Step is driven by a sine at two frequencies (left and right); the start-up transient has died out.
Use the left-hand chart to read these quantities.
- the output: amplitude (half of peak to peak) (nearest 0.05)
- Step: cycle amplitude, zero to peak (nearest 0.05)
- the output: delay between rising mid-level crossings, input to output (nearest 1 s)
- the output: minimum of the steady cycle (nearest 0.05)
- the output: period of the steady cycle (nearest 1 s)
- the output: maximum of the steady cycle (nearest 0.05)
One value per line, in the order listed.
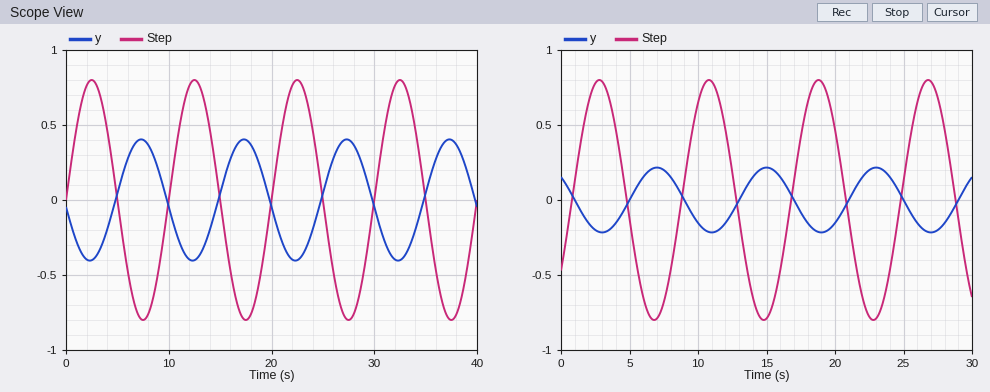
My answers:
0.40
0.80
5 s
-0.40
10 s
0.40
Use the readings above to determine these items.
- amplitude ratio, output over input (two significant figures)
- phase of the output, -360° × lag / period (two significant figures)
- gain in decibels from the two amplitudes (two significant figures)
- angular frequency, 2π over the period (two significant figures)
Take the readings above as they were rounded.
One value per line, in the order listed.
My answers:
0.50
-180°
-6.0 dB
0.63 rad/s
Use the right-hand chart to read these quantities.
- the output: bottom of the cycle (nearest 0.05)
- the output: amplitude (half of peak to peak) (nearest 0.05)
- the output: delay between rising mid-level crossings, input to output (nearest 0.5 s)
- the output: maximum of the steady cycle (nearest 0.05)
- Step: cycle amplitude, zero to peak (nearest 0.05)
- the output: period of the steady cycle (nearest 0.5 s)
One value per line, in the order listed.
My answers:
-0.20
0.20
4.0 s
0.20
0.80
8.0 s
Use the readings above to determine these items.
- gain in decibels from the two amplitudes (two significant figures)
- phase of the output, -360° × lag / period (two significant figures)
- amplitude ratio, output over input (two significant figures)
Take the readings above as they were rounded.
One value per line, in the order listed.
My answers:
-12 dB
-180°
0.25
